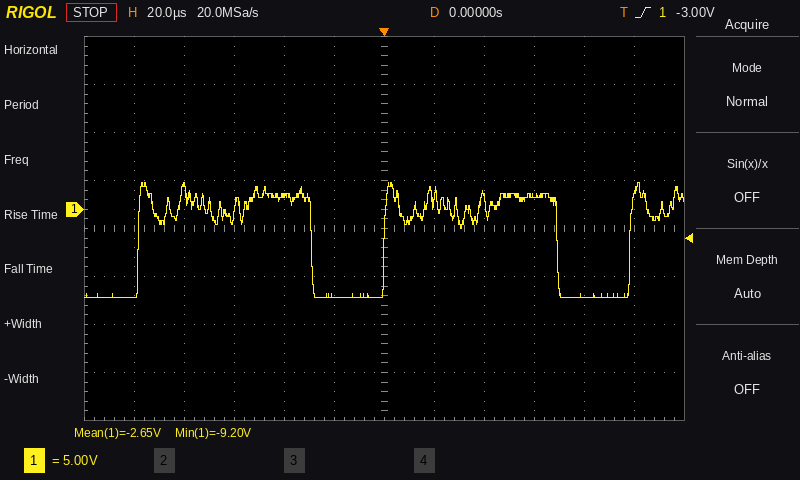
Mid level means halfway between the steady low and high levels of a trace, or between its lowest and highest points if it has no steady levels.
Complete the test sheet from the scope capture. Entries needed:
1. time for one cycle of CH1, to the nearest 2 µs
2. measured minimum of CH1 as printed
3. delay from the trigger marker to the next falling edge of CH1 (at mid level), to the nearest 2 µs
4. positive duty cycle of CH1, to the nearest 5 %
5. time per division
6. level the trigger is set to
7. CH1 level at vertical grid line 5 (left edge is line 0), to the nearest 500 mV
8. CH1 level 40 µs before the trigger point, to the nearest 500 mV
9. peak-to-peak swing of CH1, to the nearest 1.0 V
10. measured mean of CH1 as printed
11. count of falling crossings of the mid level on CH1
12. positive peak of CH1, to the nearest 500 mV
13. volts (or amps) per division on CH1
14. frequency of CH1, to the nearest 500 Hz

98 µs
-9.20 V
70 µs
70 %
20 µs
-3.00 V
-9.0 V
1.5 V
12.0 V
-2.65 V
2
3.0 V
5 V
10.0 kHz
